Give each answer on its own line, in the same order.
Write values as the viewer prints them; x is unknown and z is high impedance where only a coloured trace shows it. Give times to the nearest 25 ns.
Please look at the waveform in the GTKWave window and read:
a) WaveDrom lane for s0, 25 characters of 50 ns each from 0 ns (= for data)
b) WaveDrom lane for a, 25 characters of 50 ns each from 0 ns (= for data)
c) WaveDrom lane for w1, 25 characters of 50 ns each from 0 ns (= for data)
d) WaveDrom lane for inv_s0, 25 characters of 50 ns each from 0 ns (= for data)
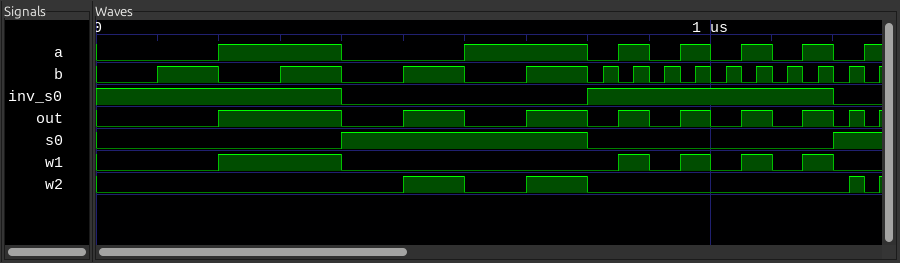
{name: 's0', wave: '0.......1.......0.......1'}
{name: 'a', wave: '0...1...0...1...010101010'}
{name: 'w1', wave: '0...1...0........10101010'}
{name: 'inv_s0', wave: '1.......0.......1.......0'}
